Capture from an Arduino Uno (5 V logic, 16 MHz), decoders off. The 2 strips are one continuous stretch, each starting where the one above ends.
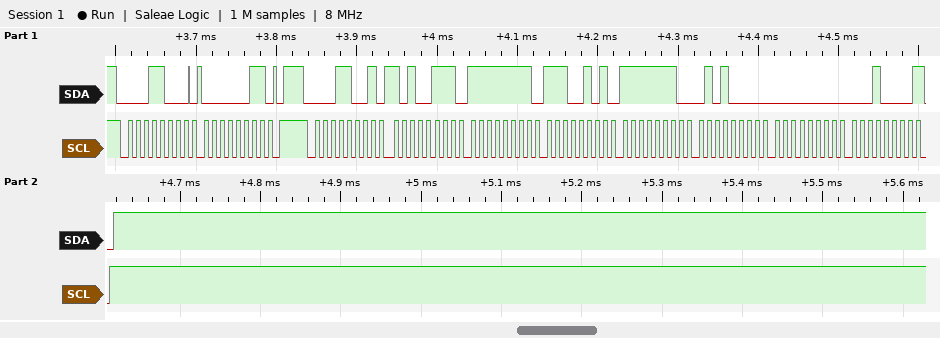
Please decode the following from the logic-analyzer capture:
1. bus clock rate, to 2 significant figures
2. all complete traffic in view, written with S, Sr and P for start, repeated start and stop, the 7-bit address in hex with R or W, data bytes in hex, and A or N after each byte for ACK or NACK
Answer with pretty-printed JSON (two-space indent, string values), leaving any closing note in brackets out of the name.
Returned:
{
  "bus clock rate, to 2 significant figures": "100 kHz",
  "all complete traffic in view, written with S, Sr and P for start, repeated start and stop, the 7-bit address in hex with R or W, data bytes in hex, and A or N after each byte for ACK or NACK": "S 0CW A 03 A P S 0CR A A7 A FF A E5 A FE A 50 A 00 A 10 N P"
}
